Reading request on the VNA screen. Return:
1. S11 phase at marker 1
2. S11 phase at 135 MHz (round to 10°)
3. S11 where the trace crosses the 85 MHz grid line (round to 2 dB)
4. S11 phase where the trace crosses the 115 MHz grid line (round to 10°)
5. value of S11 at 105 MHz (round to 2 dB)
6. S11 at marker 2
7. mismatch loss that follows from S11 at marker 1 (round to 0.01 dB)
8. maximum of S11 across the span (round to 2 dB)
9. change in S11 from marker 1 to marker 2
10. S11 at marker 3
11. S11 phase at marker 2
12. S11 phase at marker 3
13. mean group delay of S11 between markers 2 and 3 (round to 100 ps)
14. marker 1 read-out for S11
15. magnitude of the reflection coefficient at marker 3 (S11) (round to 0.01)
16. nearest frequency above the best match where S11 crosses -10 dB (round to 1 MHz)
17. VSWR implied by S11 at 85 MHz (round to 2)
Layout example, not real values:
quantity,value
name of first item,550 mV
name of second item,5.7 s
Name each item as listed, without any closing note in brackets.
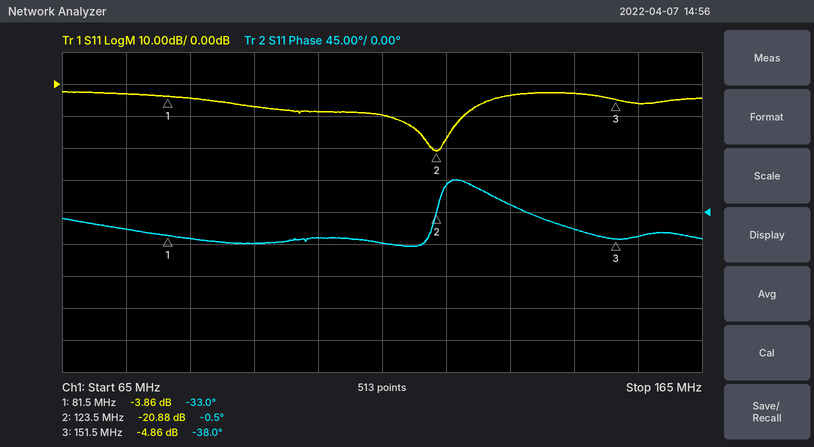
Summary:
quantity,value
S11 phase at marker 1,-33.0°
S11 phase at 135 MHz,10°
S11 where the trace crosses the 85 MHz grid line,-4 dB
S11 phase where the trace crosses the 115 MHz grid line,-40°
value of S11 at 105 MHz,-8 dB
S11 at marker 2,-20.88 dB
mismatch loss that follows from S11 at marker 1,2.30 dB
maximum of S11 across the span,-2 dB
change in S11 from marker 1 to marker 2,-17.02 dB
S11 at marker 3,-4.86 dB
S11 phase at marker 2,-0.5°
S11 phase at marker 3,-38.0°
mean group delay of S11 between markers 2 and 3,3.7 ns
marker 1 read-out for S11,-3.86 dB
magnitude of the reflection coefficient at marker 3 (S11),0.57
nearest frequency above the best match where S11 crosses -10 dB,128 MHz
VSWR implied by S11 at 85 MHz,4
